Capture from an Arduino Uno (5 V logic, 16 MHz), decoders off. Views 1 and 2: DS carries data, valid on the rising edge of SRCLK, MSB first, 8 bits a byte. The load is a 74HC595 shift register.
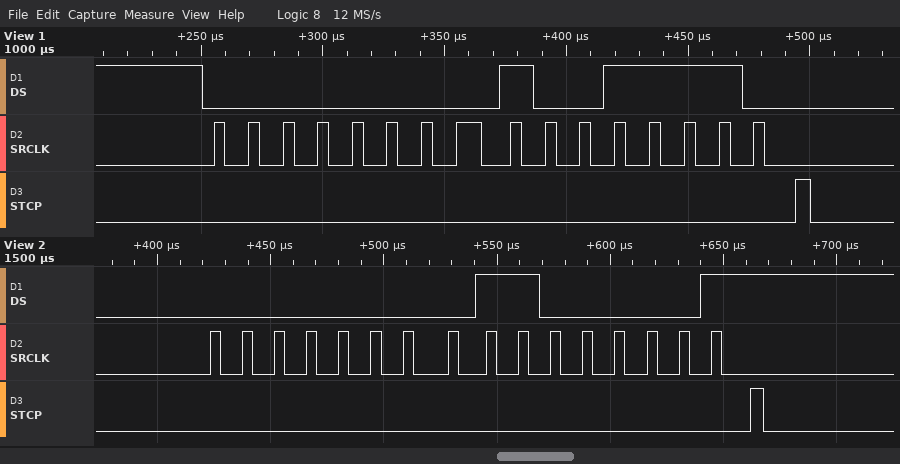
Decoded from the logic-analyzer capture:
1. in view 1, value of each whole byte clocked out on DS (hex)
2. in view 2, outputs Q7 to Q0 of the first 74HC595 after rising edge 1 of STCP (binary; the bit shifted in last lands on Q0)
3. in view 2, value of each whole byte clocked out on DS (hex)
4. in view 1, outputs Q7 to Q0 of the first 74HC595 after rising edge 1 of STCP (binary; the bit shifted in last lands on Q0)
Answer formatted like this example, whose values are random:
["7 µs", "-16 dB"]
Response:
["00 9E", "11000001", "00 C1", "10011110"]
